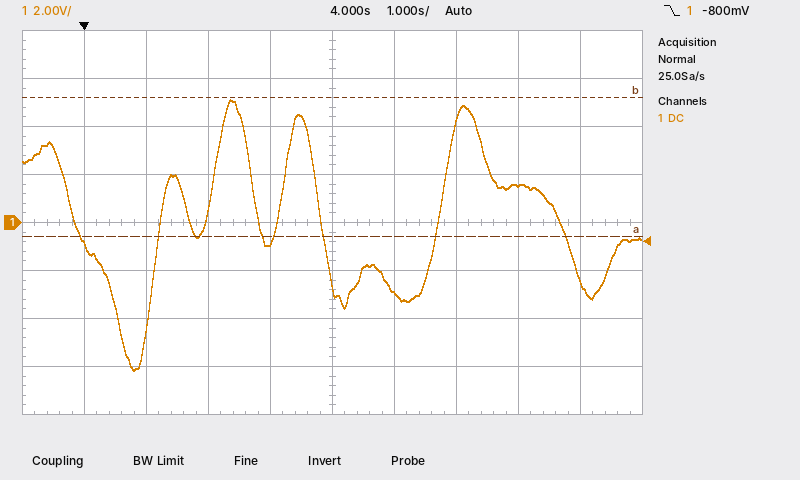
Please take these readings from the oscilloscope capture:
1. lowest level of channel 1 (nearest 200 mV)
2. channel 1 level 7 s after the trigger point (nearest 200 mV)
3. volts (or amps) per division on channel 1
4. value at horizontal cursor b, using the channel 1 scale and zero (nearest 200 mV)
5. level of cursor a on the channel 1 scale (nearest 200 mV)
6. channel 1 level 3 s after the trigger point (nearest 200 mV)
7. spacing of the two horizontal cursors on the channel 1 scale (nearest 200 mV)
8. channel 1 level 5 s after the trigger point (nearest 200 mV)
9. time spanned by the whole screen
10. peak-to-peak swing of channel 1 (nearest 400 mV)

-6.2 V
1.6 V
2 V
5.2 V
-600 mV
-800 mV
5.8 V
-3.0 V
10 s
11.2 V
